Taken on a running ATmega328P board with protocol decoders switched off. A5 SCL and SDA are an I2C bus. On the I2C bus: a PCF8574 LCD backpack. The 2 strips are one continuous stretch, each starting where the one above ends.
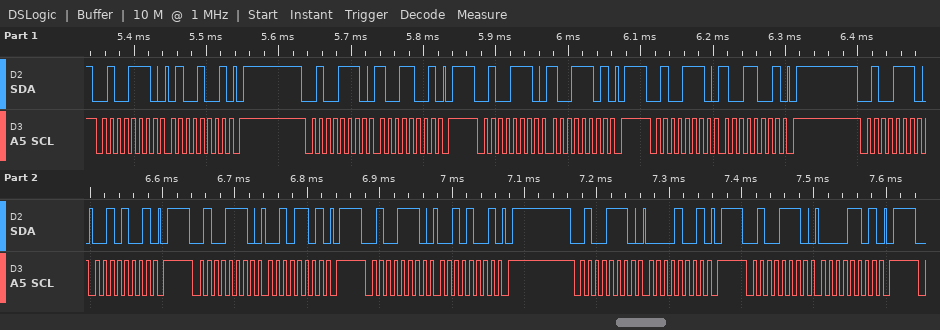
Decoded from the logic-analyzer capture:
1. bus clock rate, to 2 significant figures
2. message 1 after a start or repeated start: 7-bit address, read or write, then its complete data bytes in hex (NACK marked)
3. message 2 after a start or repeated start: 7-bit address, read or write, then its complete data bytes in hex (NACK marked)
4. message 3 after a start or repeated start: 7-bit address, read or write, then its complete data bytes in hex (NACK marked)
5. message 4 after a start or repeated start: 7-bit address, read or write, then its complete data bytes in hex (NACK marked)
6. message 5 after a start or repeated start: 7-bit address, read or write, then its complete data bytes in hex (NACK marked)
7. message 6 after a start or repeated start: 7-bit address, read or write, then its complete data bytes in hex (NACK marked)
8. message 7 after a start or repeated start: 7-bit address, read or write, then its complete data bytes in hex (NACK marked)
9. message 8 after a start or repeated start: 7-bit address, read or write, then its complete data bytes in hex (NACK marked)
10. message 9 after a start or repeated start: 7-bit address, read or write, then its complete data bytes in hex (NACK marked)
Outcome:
100 kHz
0x27 write: 49
0x27 write: 99
0x27 write: 9D
0x27 write: 99
0x27 write: 29
0x27 write: 2D
0x27 write: 29
0x27 write: 09
0x27 write: 0D
